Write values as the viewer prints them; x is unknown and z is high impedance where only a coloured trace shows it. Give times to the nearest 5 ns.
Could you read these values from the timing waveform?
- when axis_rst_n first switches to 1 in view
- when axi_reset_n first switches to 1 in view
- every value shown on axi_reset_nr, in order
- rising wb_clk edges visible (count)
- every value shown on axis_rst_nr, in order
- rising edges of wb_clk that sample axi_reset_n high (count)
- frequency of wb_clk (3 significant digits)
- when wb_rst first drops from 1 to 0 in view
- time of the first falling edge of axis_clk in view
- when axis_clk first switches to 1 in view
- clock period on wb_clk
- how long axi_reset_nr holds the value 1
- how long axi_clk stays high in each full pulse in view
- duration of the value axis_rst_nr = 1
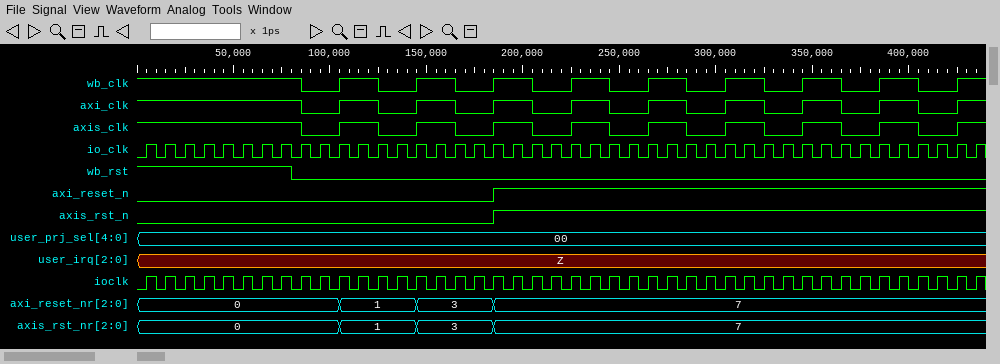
185 ns
185 ns
0, 1, 3, 7
9
0, 1, 3, 7
6
25.0 MHz
80 ns
85 ns
105 ns
40 ns
40 ns
20 ns, 20 ns, 20 ns, 20 ns, 20 ns, 20 ns, 20 ns, 20 ns
40 ns
